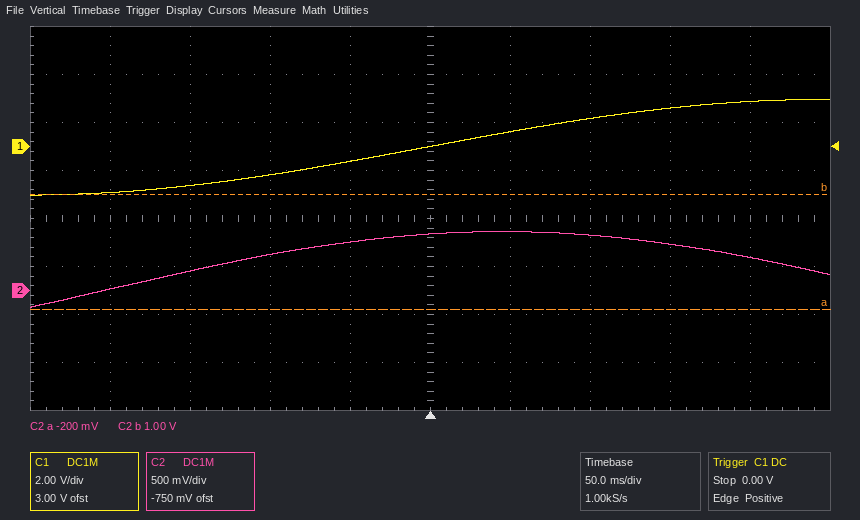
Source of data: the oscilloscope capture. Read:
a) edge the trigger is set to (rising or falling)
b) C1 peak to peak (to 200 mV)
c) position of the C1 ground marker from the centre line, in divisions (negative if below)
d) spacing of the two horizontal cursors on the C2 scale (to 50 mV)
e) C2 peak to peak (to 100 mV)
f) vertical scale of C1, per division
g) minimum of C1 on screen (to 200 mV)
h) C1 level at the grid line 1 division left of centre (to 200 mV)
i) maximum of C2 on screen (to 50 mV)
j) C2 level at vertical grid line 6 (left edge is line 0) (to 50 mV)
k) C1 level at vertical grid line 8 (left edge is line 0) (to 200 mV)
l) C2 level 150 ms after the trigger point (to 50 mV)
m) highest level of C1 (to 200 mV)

rising
4.0 V
+1.5 div
1.20 V
800 mV
2 V
-2.0 V
-600 mV
600 mV
600 mV
1.6 V
500 mV
2.0 V
